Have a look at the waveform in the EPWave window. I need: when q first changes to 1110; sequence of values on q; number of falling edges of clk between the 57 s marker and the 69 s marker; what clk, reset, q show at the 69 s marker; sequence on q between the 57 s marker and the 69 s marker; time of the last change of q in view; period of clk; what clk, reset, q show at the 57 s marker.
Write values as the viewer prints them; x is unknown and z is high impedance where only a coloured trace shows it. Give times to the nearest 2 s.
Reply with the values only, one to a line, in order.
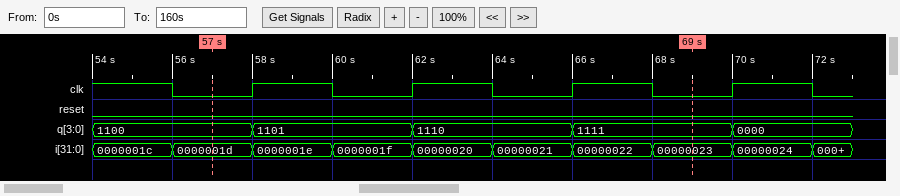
62 s
1100, 1101, 1110, 1111, 0000
3
clk=0, reset=0, q=1111
1100, 1101, 1110, 1111
70 s
4 s
clk=0, reset=0, q=1100
